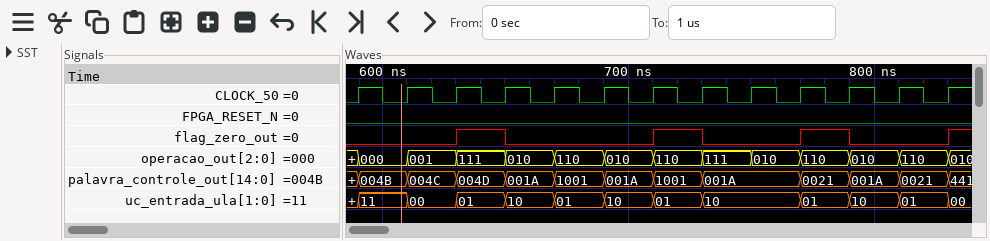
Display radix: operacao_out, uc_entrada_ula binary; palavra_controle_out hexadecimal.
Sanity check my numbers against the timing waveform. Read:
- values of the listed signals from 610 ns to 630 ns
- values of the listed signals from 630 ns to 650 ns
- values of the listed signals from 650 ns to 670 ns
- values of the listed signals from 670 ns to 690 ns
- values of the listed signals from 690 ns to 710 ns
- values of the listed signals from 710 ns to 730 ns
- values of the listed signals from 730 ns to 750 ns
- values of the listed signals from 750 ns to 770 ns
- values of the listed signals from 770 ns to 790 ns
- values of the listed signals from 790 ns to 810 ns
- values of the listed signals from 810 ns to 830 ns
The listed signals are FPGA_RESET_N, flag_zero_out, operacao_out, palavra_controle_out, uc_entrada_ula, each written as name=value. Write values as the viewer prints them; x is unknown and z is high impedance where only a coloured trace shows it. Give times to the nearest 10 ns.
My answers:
FPGA_RESET_N=0, flag_zero_out=0, operacao_out=001, palavra_controle_out=004C, uc_entrada_ula=00
FPGA_RESET_N=0, flag_zero_out=1, operacao_out=111, palavra_controle_out=004D, uc_entrada_ula=01
FPGA_RESET_N=0, flag_zero_out=0, operacao_out=010, palavra_controle_out=001A, uc_entrada_ula=10
FPGA_RESET_N=0, flag_zero_out=0, operacao_out=110, palavra_controle_out=1001, uc_entrada_ula=01
FPGA_RESET_N=0, flag_zero_out=0, operacao_out=010, palavra_controle_out=001A, uc_entrada_ula=10
FPGA_RESET_N=0, flag_zero_out=1, operacao_out=110, palavra_controle_out=1001, uc_entrada_ula=01
FPGA_RESET_N=0, flag_zero_out=0, operacao_out=111, palavra_controle_out=001A, uc_entrada_ula=10
FPGA_RESET_N=0, flag_zero_out=0, operacao_out=010, palavra_controle_out=001A, uc_entrada_ula=10
FPGA_RESET_N=0, flag_zero_out=1, operacao_out=110, palavra_controle_out=0021, uc_entrada_ula=01
FPGA_RESET_N=0, flag_zero_out=0, operacao_out=010, palavra_controle_out=001A, uc_entrada_ula=10
FPGA_RESET_N=0, flag_zero_out=0, operacao_out=110, palavra_controle_out=0021, uc_entrada_ula=01
